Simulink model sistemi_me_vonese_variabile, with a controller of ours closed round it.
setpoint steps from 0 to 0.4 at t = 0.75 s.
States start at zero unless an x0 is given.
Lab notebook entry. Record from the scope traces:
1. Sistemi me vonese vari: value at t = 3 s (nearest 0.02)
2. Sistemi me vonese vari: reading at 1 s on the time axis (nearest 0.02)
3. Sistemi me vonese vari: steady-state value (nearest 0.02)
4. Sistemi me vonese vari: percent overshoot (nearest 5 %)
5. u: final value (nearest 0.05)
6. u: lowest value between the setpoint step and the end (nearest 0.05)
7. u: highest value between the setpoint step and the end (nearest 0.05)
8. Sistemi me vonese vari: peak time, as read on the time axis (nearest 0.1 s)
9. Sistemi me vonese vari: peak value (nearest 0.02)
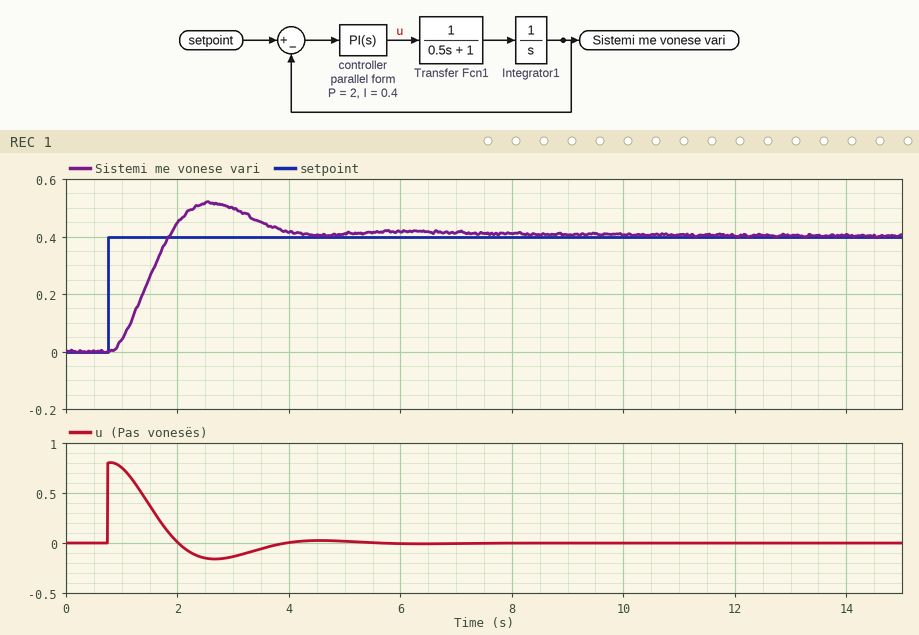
0.50
0.04
0.40
30 %
0.00
-0.15
0.80
2.6 s
0.52
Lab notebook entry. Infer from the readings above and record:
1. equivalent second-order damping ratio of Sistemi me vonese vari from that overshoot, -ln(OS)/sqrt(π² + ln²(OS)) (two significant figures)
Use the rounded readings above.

0.36
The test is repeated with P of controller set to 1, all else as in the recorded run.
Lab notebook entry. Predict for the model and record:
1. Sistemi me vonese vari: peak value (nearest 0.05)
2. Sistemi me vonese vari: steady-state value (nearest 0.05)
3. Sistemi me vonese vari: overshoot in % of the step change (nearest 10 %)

0.55
0.40
40 %
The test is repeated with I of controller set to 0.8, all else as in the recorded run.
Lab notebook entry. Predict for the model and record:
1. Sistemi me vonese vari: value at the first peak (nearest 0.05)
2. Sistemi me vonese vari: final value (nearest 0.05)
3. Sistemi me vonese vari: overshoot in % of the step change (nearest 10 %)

0.55
0.40
40 %
